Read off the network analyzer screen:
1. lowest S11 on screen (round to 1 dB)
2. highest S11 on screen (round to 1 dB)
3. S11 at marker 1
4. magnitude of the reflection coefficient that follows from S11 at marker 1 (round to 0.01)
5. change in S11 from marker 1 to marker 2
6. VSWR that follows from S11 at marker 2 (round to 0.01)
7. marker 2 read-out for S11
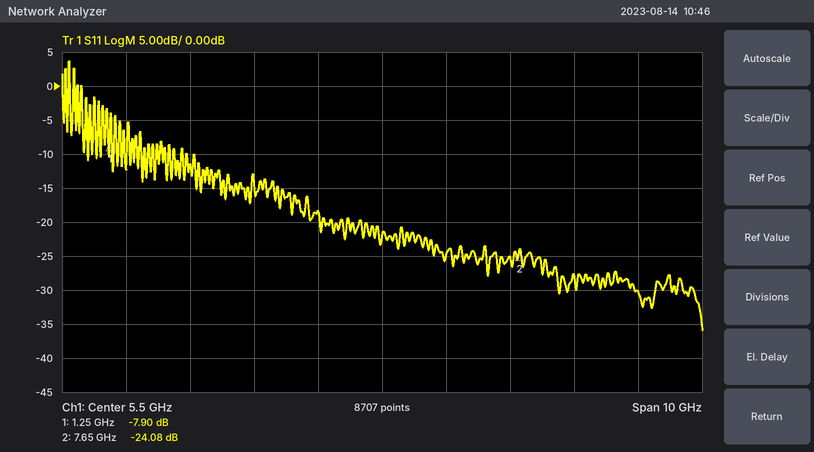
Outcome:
-36 dB
4 dB
-7.90 dB
0.40
-16.18 dB
1.13
-24.08 dB
